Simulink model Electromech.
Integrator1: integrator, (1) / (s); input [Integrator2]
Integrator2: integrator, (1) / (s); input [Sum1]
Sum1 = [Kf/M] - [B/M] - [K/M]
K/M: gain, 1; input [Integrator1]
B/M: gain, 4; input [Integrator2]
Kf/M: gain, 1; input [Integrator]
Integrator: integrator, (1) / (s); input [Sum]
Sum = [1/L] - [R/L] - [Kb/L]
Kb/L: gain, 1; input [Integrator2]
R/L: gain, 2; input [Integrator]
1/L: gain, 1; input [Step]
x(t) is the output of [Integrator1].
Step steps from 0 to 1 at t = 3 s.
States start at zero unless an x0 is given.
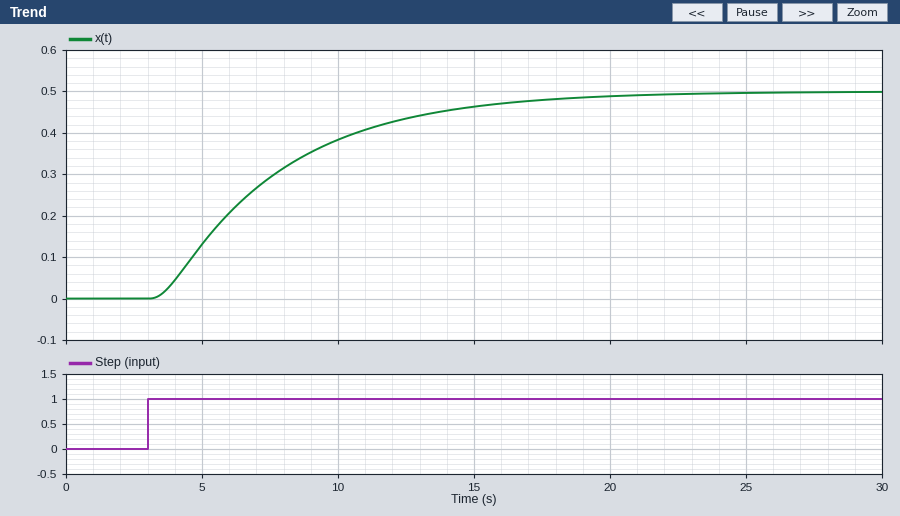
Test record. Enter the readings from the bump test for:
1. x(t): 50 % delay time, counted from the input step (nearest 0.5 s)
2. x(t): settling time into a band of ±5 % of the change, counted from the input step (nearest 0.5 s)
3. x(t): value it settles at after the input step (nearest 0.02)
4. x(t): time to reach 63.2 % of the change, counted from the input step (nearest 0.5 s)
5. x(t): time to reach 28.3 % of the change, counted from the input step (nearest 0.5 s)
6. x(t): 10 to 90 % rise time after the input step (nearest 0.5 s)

3.5 s
13.5 s
0.50
5.0 s
2.0 s
9.5 s
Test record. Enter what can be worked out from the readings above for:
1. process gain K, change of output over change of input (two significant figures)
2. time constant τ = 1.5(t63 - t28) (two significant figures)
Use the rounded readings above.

0.50
4.5 s
